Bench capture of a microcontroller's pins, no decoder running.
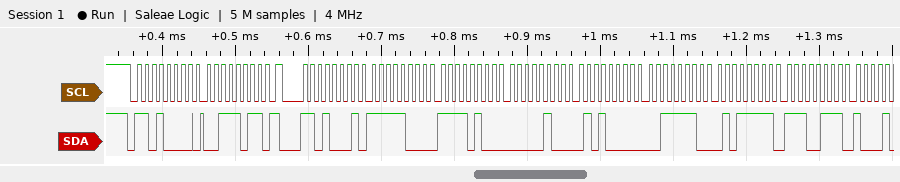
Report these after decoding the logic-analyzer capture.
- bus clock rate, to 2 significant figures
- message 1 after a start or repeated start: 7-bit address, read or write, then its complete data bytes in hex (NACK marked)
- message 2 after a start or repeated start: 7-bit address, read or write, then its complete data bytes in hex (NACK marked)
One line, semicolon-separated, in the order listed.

100 kHz; 0x68 write: 3B; 0x68 read: F8 F4 04 50 3E 5F E7
